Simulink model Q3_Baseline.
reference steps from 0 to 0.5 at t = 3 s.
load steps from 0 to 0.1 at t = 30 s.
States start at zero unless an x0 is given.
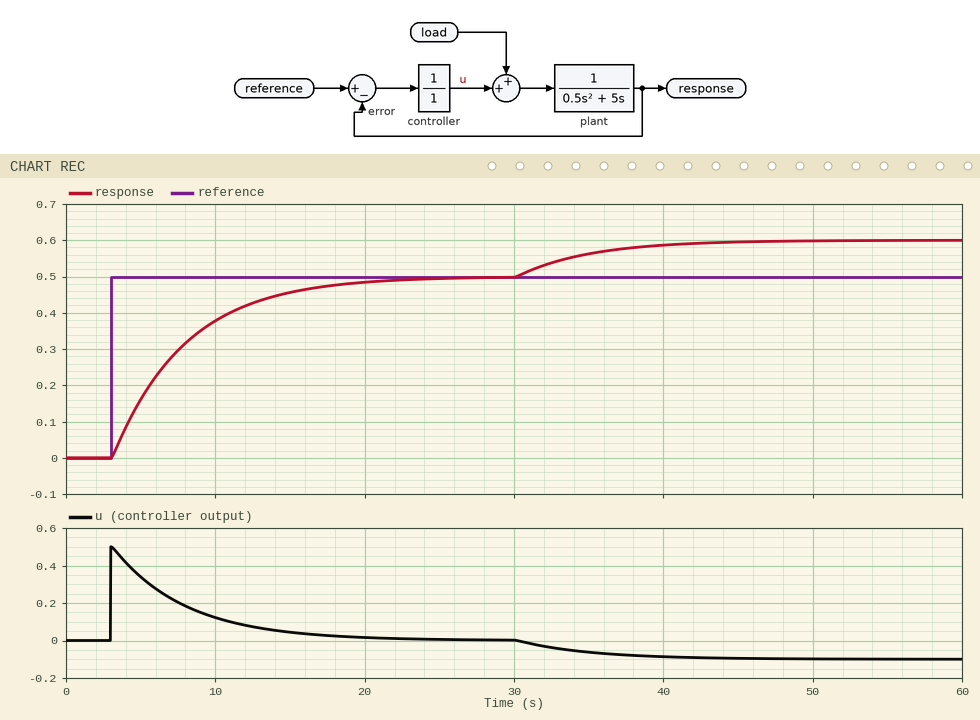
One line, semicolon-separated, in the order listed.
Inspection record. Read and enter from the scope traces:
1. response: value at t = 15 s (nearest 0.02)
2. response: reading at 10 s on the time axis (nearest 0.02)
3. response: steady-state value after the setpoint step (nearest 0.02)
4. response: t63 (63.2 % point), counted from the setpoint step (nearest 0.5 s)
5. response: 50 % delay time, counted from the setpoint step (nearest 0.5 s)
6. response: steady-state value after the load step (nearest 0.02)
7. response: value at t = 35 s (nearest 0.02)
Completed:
0.46; 0.38; 0.50; 5.0 s; 3.5 s; 0.60; 0.56
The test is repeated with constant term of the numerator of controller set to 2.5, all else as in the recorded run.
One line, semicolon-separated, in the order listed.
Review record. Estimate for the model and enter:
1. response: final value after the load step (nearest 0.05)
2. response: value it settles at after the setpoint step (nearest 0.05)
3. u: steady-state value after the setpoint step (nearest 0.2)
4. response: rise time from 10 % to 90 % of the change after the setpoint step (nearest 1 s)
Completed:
0.55; 0.50; 0.0; 4 s
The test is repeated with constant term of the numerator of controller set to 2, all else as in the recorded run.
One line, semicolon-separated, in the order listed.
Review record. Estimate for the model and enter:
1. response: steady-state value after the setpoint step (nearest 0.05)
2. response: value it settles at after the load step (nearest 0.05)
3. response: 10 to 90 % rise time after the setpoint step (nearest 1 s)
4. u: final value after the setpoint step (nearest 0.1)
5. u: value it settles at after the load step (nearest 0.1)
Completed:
0.50; 0.55; 5 s; 0.0; -0.1
